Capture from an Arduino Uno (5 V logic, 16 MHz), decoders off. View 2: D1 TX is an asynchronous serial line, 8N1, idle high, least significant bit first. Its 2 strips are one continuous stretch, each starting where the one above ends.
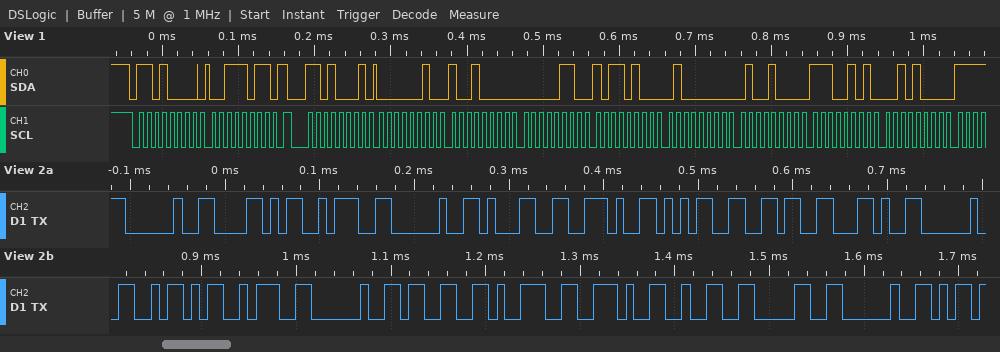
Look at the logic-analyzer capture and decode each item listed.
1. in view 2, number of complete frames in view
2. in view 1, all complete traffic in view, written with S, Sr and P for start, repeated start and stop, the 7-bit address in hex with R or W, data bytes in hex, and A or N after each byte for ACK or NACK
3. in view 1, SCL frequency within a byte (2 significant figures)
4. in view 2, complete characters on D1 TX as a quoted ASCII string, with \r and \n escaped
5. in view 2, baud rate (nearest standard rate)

19
S 68W A 3B A Sr 68R A 02 A 90 A 06 A B4 A 40 A 48 A E5 A 28 A
100 kHz
" X: 1.56, Z: 39.20 "
115200 baud
